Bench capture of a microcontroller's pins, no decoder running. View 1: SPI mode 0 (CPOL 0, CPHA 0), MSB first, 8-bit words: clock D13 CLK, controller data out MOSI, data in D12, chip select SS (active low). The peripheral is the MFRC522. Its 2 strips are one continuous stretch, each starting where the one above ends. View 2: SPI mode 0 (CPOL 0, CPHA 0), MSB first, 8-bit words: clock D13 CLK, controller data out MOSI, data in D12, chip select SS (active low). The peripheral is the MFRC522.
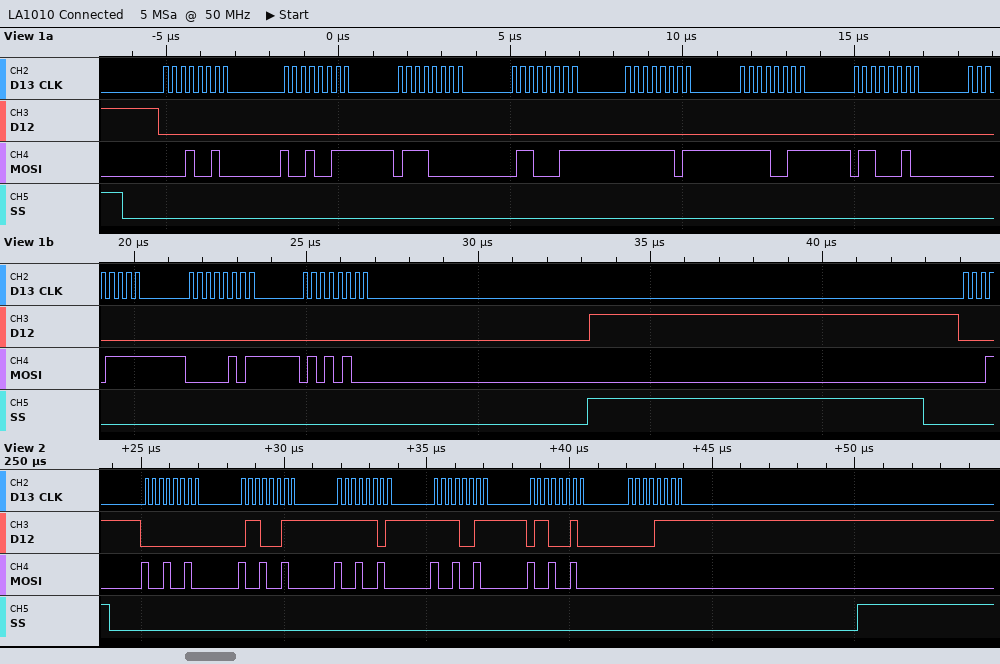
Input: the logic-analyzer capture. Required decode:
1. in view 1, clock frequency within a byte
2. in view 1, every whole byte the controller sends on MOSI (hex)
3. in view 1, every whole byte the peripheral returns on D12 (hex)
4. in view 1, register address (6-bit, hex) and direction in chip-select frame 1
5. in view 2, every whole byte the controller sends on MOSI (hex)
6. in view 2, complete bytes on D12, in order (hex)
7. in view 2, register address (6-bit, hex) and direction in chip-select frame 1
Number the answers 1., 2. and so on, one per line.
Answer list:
1. 4 MHz
2. 0x12 0x93 0x70 0x63 0xFD 0xF3 0x62 0x0F 0x05 0x54
3. 0x00 0x00 0x00 0x00 0x00 0x00 0x00 0x00 0x00 0x00
4. 0x09 write
5. 92 92 92 92 92 00
6. 00 63 FD F3 62 0F
7. 0x09 read
